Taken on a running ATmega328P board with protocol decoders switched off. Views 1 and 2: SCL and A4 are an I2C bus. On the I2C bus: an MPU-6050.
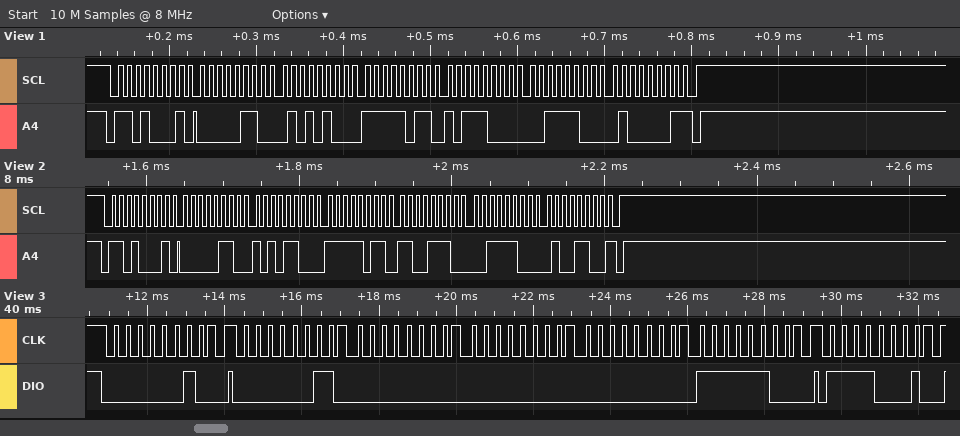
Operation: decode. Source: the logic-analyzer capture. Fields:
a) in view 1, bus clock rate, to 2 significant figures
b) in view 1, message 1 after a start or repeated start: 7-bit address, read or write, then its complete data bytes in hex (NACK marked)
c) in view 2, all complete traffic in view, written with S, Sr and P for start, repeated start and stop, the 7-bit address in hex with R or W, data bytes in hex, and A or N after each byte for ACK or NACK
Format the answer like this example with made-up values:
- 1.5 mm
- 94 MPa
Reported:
- 100 kHz
- 0x68 read: 06 54 FB B8 3C 41 NACK
- S 68R A 06 A AC A FB A CE A 3C A 4C N P
